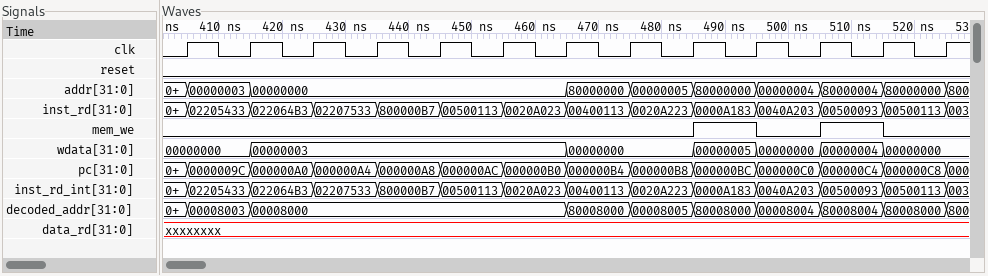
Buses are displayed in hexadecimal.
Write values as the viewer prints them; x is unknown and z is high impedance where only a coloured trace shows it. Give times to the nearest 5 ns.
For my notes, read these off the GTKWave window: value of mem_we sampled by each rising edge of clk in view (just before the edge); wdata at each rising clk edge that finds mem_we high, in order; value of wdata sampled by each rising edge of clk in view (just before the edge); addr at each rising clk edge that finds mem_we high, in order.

0 0 0 0 0 0 0 0 0 1 0 1 0
00000005, 00000004
00000000, 00000000, 00000003, 00000003, 00000003, 00000003, 00000003, 00000000, 00000000, 00000005, 00000000, 00000004, 00000000
80000000, 80000004
